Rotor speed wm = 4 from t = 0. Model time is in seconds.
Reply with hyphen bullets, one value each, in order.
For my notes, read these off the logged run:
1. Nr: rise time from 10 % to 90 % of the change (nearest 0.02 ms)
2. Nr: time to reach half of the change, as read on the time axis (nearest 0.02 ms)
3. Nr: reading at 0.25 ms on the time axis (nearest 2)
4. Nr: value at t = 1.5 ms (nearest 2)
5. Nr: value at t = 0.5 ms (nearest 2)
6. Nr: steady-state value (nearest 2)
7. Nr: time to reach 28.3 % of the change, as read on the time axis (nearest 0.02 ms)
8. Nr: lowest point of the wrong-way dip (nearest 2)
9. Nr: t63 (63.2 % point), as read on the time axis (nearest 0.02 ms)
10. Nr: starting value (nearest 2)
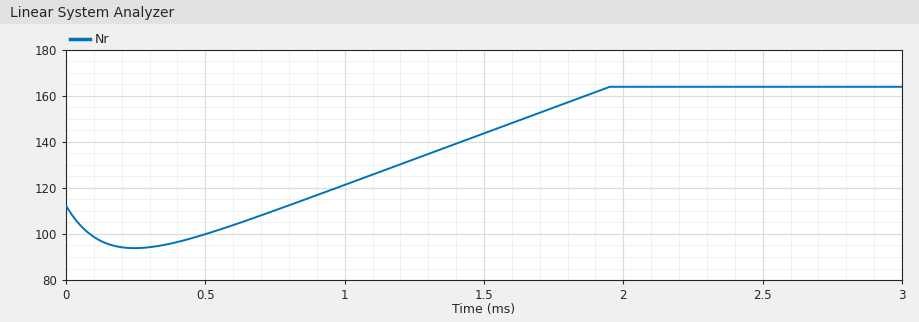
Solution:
- 0.92 ms
- 1.38 ms
- 94
- 144
- 100
- 164
- 1.12 ms
- 94
- 1.52 ms
- 112
